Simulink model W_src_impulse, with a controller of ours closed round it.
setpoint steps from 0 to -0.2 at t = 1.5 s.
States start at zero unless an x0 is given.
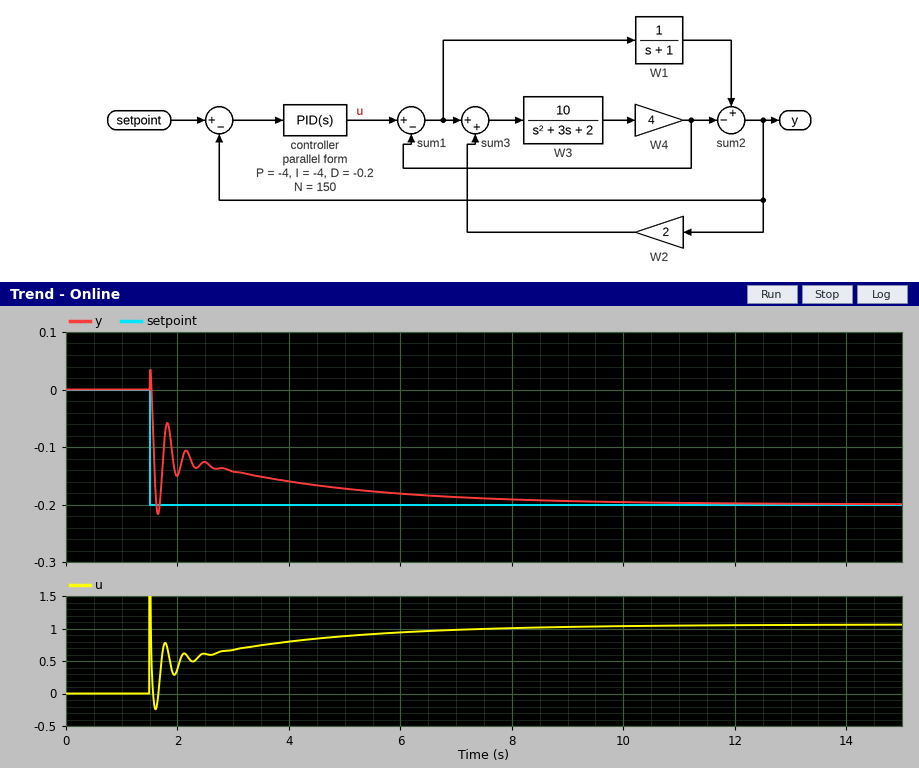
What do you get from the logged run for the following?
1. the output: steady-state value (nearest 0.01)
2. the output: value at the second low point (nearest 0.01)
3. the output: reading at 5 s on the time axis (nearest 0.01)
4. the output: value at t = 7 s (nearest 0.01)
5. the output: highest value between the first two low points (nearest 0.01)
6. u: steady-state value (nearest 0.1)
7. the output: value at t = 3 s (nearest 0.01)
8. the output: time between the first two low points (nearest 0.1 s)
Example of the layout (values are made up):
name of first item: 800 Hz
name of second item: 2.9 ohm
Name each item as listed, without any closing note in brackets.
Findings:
the output: steady-state value: -0.20
the output: value at the second low point: -0.15
the output: reading at 5 s on the time axis: -0.17
the output: value at t = 7 s: -0.19
the output: highest value between the first two low points: -0.06
u: steady-state value: 1.1
the output: value at t = 3 s: -0.14
the output: time between the first two low points: 0.3 s
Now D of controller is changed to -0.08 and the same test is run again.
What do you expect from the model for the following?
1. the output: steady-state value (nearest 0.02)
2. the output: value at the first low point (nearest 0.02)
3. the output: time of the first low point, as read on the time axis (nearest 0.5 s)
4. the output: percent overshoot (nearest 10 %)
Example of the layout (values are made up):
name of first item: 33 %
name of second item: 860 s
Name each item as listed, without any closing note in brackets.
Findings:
the output: steady-state value: -0.20
the output: value at the first low point: -0.24
the output: time of the first low point, as read on the time axis: 1.5 s
the output: percent overshoot: 20 %
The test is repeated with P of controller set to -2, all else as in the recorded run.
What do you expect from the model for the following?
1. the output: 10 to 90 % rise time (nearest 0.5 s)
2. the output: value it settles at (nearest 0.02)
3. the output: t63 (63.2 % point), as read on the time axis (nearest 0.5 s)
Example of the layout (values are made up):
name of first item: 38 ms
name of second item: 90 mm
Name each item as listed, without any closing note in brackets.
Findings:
the output: 10 to 90 % rise time: 4.0 s
the output: value it settles at: -0.20
the output: t63 (63.2 % point), as read on the time axis: 1.5 s
